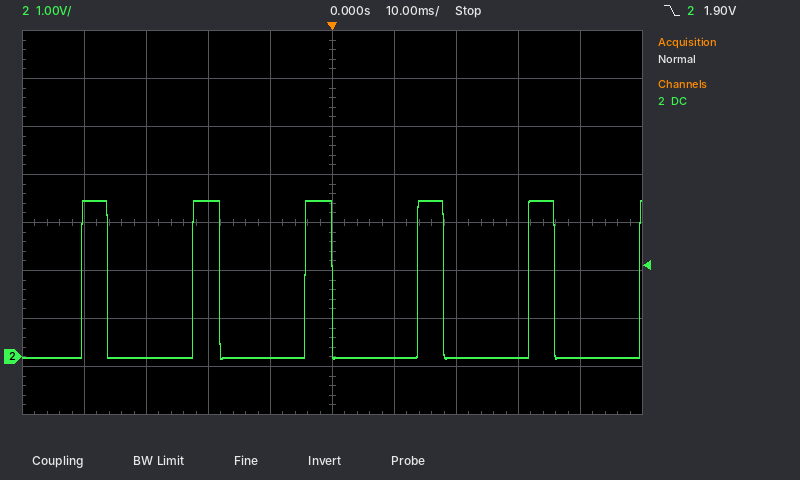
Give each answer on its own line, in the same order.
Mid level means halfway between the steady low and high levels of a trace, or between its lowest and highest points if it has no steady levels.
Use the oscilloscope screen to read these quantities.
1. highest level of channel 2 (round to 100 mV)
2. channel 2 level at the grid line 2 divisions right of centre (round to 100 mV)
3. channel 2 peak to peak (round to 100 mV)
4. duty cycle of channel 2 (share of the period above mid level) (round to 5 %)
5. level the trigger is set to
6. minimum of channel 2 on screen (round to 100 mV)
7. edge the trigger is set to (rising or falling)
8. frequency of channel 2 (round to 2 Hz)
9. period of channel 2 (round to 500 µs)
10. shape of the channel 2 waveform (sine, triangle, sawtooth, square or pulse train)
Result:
3.3 V
0.0 V
3.3 V
25 %
1.90 V
0.0 V
falling
56 Hz
18.0 ms
pulse train
